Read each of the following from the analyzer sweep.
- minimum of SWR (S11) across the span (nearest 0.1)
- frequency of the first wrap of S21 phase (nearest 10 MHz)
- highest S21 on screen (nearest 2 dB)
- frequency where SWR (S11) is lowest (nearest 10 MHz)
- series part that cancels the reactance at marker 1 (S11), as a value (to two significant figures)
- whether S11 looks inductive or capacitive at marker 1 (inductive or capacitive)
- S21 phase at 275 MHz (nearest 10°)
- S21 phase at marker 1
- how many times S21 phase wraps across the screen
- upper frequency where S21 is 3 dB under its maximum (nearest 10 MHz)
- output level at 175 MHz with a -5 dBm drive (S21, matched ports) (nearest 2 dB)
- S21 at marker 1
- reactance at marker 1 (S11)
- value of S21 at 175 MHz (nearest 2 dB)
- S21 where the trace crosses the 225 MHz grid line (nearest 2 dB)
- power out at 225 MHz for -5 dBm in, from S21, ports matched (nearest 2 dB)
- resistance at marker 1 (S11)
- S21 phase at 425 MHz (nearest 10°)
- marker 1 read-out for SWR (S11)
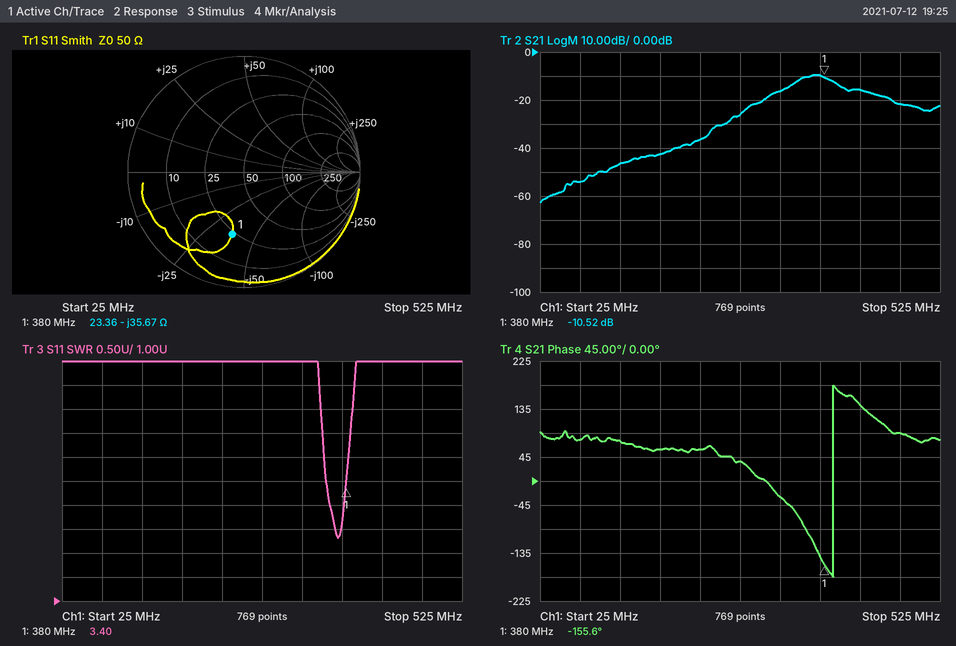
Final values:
2.3
390 MHz
-10 dB
370 MHz
15 nH
capacitive
40°
-155.6°
1
390 MHz
-48 dBm
-10.52 dB
-35.67 Ω
-42 dB
-36 dB
-42 dBm
23.36 Ω
140°
3.40
